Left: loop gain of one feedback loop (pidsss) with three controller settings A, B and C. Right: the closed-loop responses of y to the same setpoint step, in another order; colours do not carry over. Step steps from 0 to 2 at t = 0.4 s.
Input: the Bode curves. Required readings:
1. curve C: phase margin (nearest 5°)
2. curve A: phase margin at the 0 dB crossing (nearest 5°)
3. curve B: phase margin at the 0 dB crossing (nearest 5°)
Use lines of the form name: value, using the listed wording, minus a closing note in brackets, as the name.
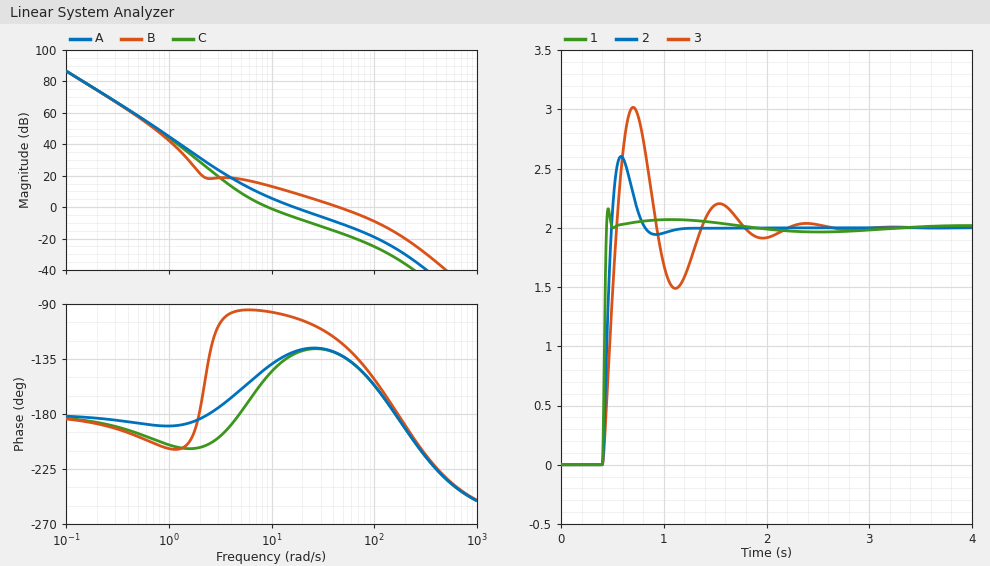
curve C: phase margin: 30°
curve A: phase margin at the 0 dB crossing: 50°
curve B: phase margin at the 0 dB crossing: 60°
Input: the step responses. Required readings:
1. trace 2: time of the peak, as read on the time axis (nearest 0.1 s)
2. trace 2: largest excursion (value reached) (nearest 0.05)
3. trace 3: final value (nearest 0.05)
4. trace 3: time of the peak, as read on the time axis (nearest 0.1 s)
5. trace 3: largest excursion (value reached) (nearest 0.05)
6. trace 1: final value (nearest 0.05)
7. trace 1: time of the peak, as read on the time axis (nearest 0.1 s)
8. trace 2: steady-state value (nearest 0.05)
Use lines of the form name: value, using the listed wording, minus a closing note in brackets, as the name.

trace 2: time of the peak, as read on the time axis: 0.6 s
trace 2: largest excursion (value reached): 2.60
trace 3: final value: 2.00
trace 3: time of the peak, as read on the time axis: 0.7 s
trace 3: largest excursion (value reached): 3.00
trace 1: final value: 2.00
trace 1: time of the peak, as read on the time axis: 0.5 s
trace 2: steady-state value: 2.00
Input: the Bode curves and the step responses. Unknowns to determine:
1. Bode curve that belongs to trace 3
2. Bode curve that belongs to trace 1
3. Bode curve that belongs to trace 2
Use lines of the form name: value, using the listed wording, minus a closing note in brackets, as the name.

Bode curve that belongs to trace 3: C
Bode curve that belongs to trace 1: B
Bode curve that belongs to trace 2: A
